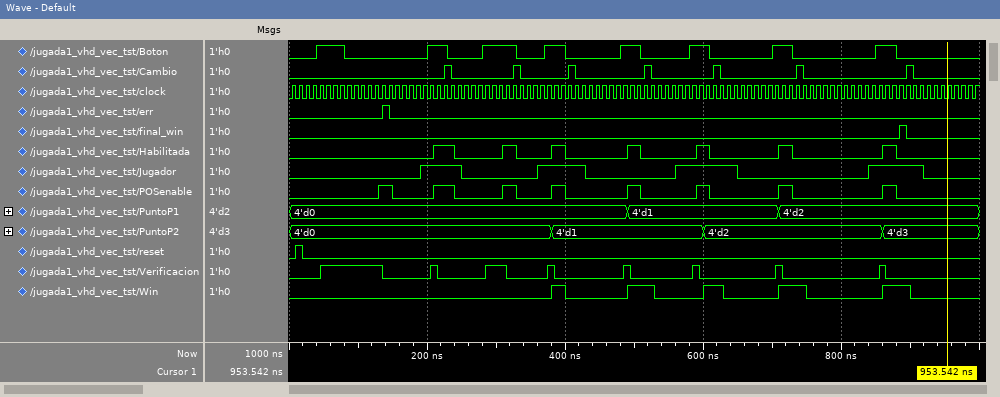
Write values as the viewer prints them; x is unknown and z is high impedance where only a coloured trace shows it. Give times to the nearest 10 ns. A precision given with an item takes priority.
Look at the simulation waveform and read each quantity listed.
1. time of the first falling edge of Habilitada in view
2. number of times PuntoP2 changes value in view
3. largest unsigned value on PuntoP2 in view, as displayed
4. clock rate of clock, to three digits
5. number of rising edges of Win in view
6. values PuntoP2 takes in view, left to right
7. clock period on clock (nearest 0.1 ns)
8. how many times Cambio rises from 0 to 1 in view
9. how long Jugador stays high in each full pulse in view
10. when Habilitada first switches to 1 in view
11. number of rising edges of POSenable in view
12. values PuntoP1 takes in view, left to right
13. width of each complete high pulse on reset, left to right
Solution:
240 ns
3
4'd3
100 MHz
5
4'd0, 4'd1, 4'd2, 4'd3
10 ns
7
60 ns, 70 ns, 90 ns, 80 ns
210 ns
8
4'd0, 4'd1, 4'd2
10 ns
